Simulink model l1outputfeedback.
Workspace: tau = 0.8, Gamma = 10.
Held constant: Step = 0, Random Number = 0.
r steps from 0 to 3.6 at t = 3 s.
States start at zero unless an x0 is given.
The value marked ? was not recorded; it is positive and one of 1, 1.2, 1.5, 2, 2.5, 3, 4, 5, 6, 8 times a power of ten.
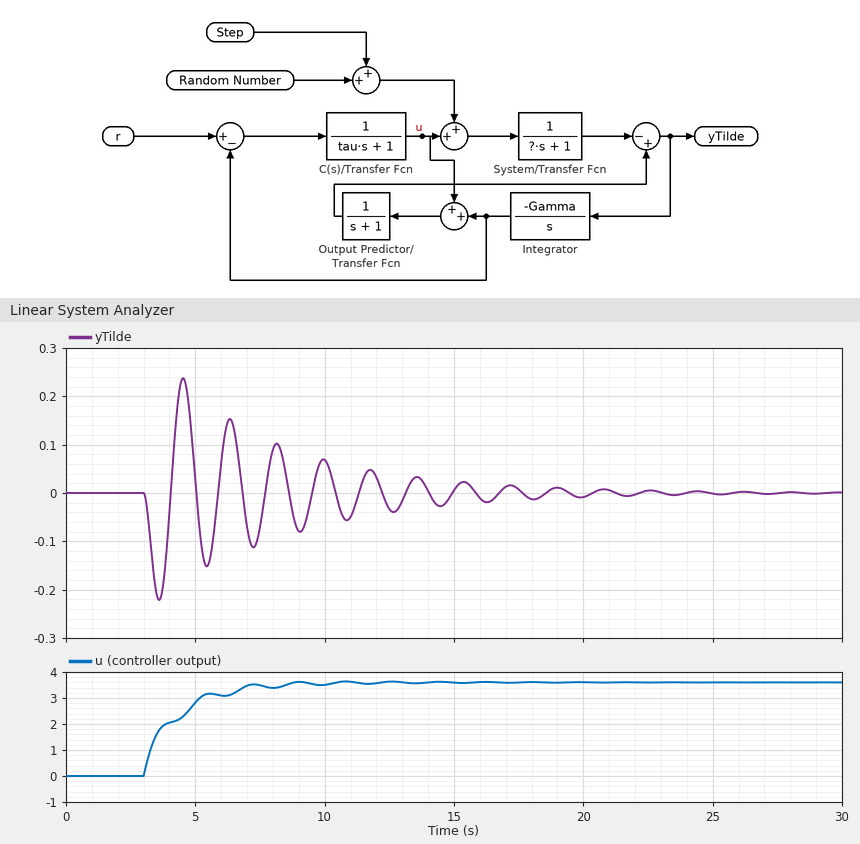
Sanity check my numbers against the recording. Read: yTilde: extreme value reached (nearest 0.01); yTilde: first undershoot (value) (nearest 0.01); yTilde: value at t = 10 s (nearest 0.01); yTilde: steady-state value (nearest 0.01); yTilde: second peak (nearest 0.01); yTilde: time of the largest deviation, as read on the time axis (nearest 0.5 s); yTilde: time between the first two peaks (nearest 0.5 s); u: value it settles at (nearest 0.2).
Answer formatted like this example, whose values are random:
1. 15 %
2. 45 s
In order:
1. 0.24
2. -0.15
3. 0.07
4. 0.00
5. 0.15
6. 4.5 s
7. 2.0 s
8. 3.6
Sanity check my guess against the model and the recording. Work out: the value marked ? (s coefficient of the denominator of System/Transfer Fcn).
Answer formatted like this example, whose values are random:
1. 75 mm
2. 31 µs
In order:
1. 0.5
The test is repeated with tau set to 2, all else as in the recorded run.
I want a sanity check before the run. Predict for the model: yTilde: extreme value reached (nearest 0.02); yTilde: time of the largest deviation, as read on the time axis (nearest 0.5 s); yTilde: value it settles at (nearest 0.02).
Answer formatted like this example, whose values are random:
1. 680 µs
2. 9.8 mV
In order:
1. -0.12
2. 3.5 s
3. 0.00
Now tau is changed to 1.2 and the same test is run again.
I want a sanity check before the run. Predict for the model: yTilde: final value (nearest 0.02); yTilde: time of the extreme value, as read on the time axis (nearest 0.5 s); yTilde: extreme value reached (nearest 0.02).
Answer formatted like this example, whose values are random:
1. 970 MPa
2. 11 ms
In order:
1. 0.00
2. 3.5 s
3. -0.16
